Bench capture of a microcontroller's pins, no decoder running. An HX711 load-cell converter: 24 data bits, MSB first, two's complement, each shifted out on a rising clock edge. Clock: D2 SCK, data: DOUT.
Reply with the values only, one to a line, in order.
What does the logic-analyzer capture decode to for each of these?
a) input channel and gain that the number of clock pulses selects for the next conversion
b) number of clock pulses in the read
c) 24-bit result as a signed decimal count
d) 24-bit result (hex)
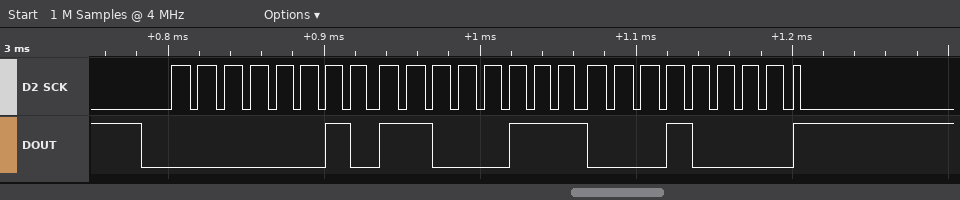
channel A, gain 128
25
182032
0x02C710
